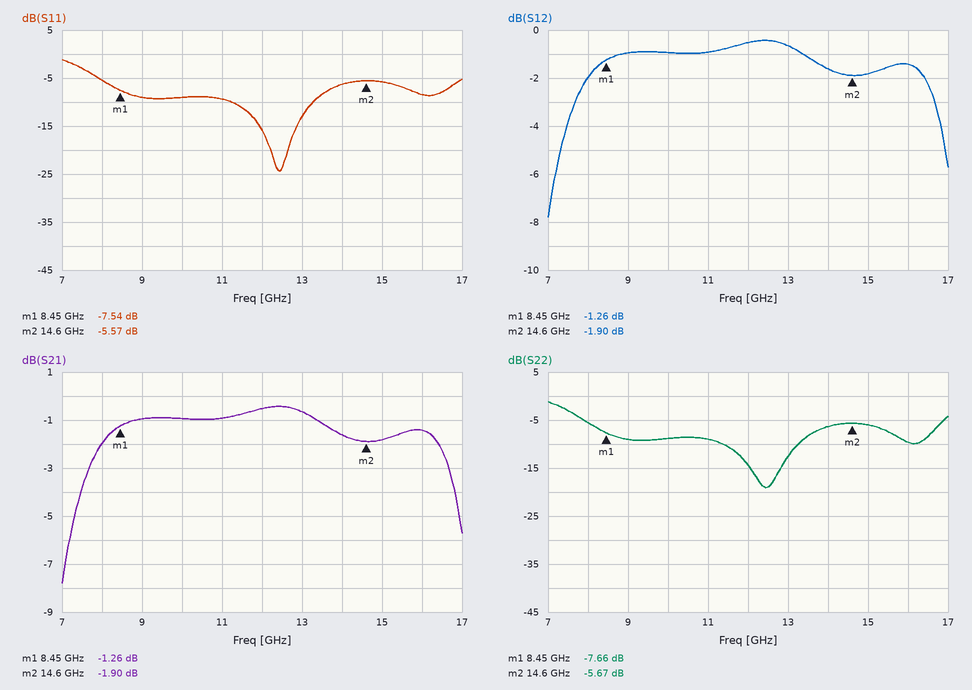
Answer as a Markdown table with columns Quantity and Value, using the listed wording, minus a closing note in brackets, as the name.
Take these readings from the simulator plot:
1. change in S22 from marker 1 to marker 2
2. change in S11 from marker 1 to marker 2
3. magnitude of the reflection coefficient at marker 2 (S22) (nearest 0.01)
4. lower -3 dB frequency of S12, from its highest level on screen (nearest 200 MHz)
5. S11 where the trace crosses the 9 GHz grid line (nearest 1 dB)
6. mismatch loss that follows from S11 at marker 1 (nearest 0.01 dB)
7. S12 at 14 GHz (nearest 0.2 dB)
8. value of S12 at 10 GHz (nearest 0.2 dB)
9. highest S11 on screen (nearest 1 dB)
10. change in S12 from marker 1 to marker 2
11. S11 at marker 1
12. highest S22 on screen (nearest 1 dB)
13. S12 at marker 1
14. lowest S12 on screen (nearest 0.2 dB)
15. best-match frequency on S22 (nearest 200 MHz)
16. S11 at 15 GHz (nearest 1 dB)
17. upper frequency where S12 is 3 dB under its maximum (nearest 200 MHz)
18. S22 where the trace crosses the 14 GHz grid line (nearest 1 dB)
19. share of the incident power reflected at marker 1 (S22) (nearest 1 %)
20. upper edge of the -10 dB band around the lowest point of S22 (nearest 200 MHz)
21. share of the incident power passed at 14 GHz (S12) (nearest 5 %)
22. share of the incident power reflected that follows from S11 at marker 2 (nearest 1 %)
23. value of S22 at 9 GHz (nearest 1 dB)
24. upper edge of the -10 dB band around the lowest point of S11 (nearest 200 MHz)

| Quantity | Value |
|---|---|
| change in S22 from marker 1 to marker 2 | 1.99 dB |
| change in S11 from marker 1 to marker 2 | 1.97 dB |
| magnitude of the reflection coefficient at marker 2 (S22) | 0.52 |
| lower -3 dB frequency of S12, from its highest level on screen | 7.6 GHz |
| S11 where the trace crosses the 9 GHz grid line | -9 dB |
| mismatch loss that follows from S11 at marker 1 | 0.84 dB |
| S12 at 14 GHz | -1.6 dB |
| value of S12 at 10 GHz | -1.0 dB |
| highest S11 on screen | -1 dB |
| change in S12 from marker 1 to marker 2 | -0.64 dB |
| S11 at marker 1 | -7.54 dB |
| highest S22 on screen | -1 dB |
| S12 at marker 1 | -1.26 dB |
| lowest S12 on screen | -7.8 dB |
| best-match frequency on S22 | 12.4 GHz |
| S11 at 15 GHz | -6 dB |
| upper frequency where S12 is 3 dB under its maximum | 16.8 GHz |
| S22 where the trace crosses the 14 GHz grid line | -6 dB |
| share of the incident power reflected at marker 1 (S22) | 17 % |
| upper edge of the -10 dB band around the lowest point of S22 | 13.2 GHz |
| share of the incident power passed at 14 GHz (S12) | 70 % |
| share of the incident power reflected that follows from S11 at marker 2 | 28 % |
| value of S22 at 9 GHz | -9 dB |
| upper edge of the -10 dB band around the lowest point of S11 | 13.2 GHz |
